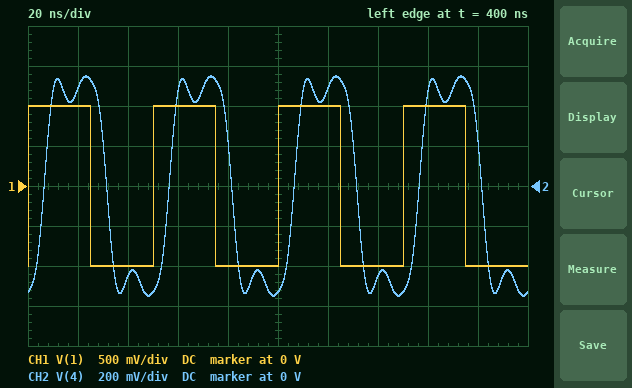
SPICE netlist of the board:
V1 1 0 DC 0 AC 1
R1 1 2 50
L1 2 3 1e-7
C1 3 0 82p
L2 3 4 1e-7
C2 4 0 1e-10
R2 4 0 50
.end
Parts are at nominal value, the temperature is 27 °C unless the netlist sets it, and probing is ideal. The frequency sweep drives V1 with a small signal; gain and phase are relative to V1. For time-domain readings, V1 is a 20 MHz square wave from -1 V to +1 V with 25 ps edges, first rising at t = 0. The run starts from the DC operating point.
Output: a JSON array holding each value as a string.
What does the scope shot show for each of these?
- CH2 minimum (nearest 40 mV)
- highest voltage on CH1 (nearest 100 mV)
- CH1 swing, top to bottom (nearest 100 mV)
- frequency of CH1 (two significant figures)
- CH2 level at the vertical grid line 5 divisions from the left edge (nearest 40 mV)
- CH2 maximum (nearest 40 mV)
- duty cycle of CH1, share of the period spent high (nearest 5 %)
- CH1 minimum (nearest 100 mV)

["-560 mV", "1.0 V", "2.0 V", "20 MHz", "-520 mV", "560 mV", "50 %", "-1.0 V"]
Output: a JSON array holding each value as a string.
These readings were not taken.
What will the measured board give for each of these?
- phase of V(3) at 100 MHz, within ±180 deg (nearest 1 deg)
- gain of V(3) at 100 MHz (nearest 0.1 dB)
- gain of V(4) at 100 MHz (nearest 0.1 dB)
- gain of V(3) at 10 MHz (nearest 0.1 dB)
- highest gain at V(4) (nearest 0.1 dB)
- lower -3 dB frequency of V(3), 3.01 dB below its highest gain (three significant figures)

["-117 deg", "-5.5 dB", "-15.6 dB", "-6.4 dB", "-6.0 dB", "71.2 MHz"]
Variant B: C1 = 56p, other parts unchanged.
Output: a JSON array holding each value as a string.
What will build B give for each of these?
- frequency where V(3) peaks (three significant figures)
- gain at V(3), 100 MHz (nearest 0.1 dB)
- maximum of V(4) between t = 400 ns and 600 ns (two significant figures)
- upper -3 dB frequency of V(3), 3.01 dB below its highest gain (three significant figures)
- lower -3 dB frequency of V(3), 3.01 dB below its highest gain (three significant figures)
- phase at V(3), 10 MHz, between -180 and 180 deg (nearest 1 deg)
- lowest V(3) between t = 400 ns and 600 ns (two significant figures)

["96.1 MHz", "1.2 dB", "560 mV", "110 MHz", "83.2 MHz", "-14 deg", "-700 mV"]
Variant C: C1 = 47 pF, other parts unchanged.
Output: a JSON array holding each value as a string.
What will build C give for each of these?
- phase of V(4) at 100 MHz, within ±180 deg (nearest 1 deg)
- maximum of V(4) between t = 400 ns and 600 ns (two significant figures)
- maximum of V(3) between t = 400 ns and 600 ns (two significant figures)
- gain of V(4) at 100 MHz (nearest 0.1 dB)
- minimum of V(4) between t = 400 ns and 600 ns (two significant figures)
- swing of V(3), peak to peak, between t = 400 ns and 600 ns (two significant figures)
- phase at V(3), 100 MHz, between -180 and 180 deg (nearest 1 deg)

["156 deg", "560 mV", "720 mV", "-8.0 dB", "-560 mV", "1.4 V", "-47 deg"]
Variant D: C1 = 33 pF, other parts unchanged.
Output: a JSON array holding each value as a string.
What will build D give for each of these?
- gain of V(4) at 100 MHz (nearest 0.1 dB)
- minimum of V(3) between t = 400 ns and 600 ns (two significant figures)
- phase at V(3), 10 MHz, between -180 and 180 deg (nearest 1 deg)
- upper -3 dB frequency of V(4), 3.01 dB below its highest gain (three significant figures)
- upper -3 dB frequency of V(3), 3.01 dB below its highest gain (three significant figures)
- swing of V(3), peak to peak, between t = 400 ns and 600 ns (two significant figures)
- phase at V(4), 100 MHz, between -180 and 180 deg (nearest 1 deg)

["-10.9 dB", "-690 mV", "-12 deg", "55.3 MHz", "138 MHz", "1.4 V", "-164 deg"]
